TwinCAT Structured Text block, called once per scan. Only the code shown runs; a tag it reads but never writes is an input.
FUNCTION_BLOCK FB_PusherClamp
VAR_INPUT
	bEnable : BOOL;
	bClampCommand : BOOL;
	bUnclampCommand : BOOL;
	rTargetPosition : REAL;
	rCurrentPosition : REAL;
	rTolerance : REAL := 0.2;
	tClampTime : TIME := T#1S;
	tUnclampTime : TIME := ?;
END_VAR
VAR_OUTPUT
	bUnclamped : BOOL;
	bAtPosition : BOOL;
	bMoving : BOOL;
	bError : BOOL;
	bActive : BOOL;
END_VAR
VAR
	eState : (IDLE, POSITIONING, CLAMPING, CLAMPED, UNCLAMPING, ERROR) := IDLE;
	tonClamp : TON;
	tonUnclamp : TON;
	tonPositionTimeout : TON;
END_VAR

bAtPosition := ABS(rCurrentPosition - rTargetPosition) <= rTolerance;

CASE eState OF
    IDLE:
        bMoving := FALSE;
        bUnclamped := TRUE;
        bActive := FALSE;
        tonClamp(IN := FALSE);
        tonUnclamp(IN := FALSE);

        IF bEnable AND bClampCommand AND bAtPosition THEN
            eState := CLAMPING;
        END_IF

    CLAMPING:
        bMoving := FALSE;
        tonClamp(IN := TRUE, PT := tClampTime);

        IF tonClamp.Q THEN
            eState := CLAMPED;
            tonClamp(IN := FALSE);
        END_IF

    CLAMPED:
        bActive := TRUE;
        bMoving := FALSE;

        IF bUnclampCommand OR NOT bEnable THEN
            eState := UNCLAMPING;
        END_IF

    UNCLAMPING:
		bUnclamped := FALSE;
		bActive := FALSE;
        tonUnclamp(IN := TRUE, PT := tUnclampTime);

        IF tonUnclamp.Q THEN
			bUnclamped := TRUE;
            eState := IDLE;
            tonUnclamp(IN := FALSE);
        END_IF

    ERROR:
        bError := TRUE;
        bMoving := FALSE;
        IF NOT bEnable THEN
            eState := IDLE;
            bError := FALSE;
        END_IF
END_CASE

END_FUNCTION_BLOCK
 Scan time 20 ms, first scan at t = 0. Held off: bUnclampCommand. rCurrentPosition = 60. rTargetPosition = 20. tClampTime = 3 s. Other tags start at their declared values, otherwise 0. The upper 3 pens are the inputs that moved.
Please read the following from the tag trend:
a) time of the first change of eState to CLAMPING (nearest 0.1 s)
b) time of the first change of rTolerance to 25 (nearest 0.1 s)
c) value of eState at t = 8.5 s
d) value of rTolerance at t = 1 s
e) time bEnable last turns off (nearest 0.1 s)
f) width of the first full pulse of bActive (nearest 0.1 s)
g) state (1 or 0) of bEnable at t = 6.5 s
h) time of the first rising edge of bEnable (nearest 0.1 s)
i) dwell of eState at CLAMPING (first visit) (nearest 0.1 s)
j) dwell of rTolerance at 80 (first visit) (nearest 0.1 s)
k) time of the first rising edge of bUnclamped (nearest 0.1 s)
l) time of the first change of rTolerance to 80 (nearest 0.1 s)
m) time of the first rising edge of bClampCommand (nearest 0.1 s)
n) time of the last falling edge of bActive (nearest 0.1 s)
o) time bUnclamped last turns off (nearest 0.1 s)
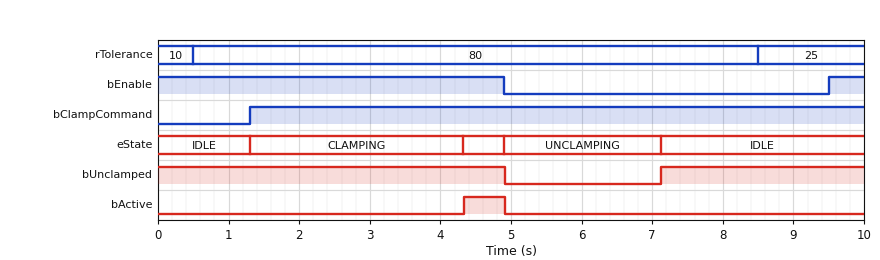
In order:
1.3 s
8.5 s
IDLE
80
4.9 s
0.6 s
0
9.5 s
3.0 s
8.0 s
7.1 s
0.5 s
1.3 s
4.9 s
4.9 s
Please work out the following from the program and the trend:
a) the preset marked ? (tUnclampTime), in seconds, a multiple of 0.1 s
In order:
2.2 s
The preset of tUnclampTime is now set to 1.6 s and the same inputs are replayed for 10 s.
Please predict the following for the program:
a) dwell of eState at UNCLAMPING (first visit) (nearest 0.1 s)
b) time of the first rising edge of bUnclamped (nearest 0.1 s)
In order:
1.6 s
6.5 s
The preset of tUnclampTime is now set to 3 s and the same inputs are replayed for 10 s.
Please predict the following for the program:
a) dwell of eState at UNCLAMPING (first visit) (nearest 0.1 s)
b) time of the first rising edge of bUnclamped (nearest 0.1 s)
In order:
3.0 s
7.9 s
